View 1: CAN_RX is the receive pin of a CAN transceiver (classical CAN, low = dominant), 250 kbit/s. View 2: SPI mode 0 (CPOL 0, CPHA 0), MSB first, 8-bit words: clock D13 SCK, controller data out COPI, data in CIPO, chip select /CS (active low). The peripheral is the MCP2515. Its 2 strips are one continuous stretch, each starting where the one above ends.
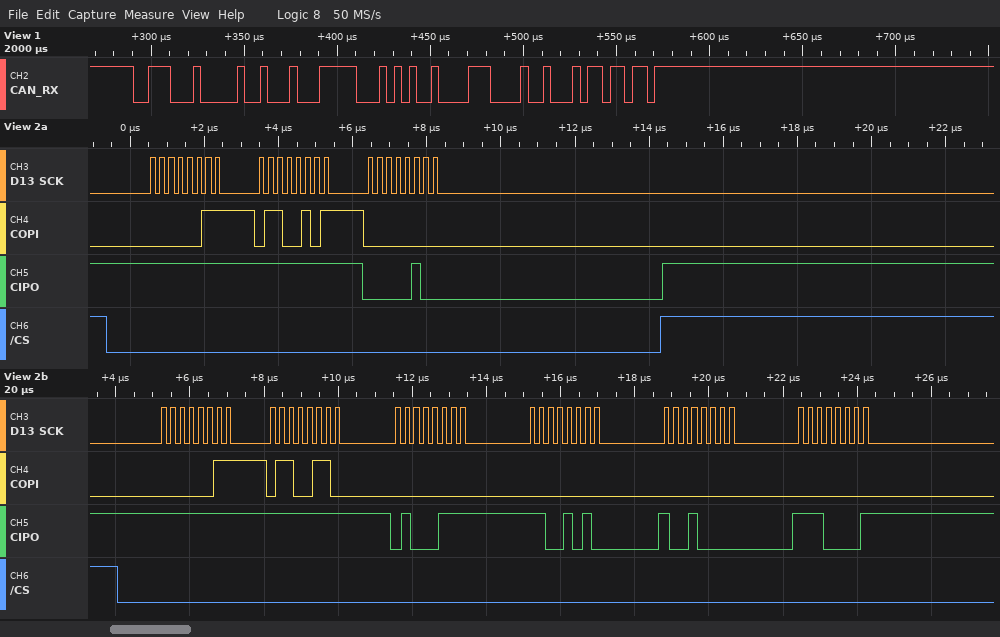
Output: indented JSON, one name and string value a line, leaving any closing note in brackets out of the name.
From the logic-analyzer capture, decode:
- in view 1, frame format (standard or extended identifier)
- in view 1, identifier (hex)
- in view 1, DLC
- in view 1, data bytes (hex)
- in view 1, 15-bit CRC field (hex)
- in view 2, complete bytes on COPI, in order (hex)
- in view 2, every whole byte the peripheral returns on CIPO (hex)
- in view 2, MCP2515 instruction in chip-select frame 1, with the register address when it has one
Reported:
{
  "in view 1, frame format": "standard",
  "in view 1, identifier": "0x388",
  "in view 1, DLC": "4",
  "in view 1, data bytes": "47 CA 90 E1",
  "in view 1, 15-bit CRC field": "0x116D",
  "in view 2, complete bytes on COPI, in order": "03 65 00 03 66 00 00 00 00",
  "in view 2, every whole byte the peripheral returns on CIPO": "FF FF 04 FF FF 47 CA 90 E1",
  "in view 2, MCP2515 instruction in chip-select frame 1, with the register address when it has one": "READ 0x65"
}
